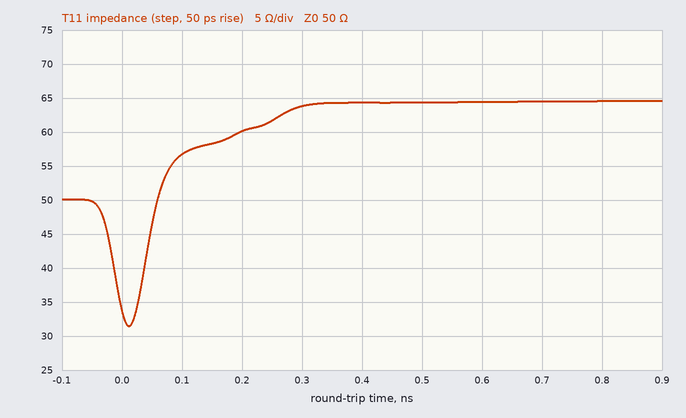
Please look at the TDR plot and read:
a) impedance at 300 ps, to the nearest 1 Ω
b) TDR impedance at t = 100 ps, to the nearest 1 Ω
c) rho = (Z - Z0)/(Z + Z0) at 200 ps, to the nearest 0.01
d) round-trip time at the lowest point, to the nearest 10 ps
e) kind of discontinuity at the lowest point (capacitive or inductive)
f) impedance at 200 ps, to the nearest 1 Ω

64 Ω
57 Ω
+0.09
10 ps
capacitive
60 Ω
